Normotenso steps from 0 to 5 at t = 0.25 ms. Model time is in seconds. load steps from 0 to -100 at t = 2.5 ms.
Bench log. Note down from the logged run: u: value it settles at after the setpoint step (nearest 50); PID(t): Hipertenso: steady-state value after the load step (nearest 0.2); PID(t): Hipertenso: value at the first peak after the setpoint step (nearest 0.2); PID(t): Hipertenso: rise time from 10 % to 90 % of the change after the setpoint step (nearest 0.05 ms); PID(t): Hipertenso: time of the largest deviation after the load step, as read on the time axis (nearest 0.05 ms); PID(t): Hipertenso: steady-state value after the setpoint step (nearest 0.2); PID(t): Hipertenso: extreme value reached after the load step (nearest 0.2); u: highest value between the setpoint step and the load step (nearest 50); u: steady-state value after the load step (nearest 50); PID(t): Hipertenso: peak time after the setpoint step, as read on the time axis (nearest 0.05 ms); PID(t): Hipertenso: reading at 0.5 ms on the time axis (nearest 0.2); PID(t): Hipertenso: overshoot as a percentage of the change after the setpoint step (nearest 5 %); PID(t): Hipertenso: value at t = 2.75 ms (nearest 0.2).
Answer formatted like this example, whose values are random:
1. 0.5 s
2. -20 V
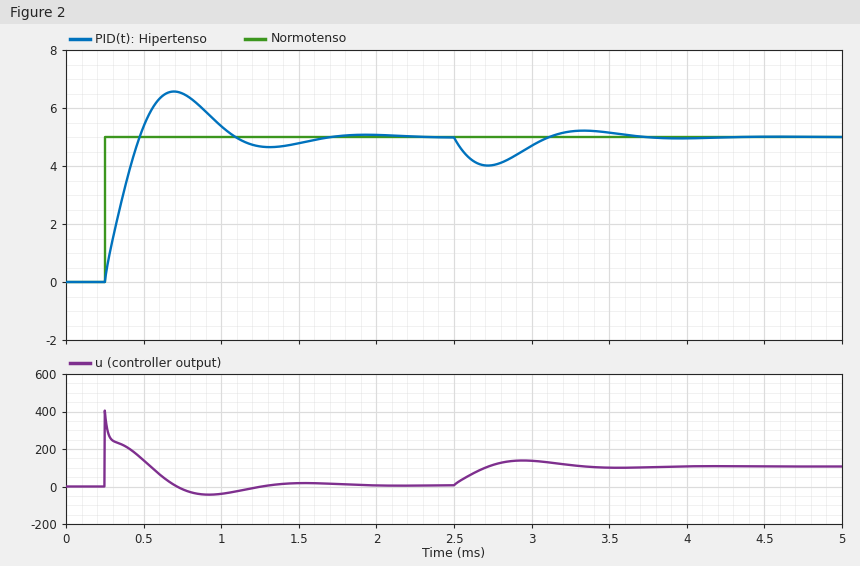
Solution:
1. 0
2. 5.0
3. 6.6
4. 0.20 ms
5. 2.70 ms
6. 5.0
7. 4.0
8. 400
9. 100
10. 0.70 ms
11. 5.4
12. 30 %
13. 4.0
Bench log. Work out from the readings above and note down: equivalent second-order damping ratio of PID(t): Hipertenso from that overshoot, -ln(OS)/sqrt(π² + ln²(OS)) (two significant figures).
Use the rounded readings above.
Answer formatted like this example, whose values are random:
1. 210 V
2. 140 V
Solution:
1. 0.36
